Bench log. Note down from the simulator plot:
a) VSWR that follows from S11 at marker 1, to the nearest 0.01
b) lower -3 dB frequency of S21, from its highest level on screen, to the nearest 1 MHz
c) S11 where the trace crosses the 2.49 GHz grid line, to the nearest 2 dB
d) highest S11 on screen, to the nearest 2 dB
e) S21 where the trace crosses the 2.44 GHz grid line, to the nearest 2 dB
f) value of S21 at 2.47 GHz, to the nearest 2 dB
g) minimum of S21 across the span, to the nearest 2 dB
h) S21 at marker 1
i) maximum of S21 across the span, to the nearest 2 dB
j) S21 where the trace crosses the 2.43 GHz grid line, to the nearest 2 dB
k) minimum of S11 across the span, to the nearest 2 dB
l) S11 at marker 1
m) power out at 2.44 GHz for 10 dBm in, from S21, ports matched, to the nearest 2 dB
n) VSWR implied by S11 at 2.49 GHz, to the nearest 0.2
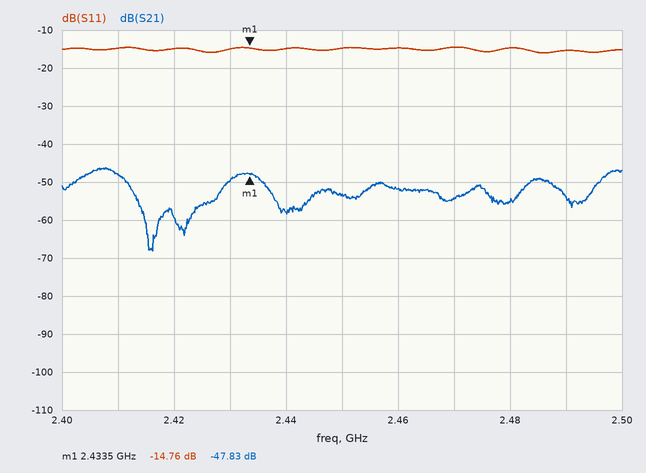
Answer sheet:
1.45
2.403 GHz
-16 dB
-14 dB
-58 dB
-54 dB
-68 dB
-47.83 dB
-46 dB
-50 dB
-16 dB
-14.76 dB
-48 dBm
1.4
